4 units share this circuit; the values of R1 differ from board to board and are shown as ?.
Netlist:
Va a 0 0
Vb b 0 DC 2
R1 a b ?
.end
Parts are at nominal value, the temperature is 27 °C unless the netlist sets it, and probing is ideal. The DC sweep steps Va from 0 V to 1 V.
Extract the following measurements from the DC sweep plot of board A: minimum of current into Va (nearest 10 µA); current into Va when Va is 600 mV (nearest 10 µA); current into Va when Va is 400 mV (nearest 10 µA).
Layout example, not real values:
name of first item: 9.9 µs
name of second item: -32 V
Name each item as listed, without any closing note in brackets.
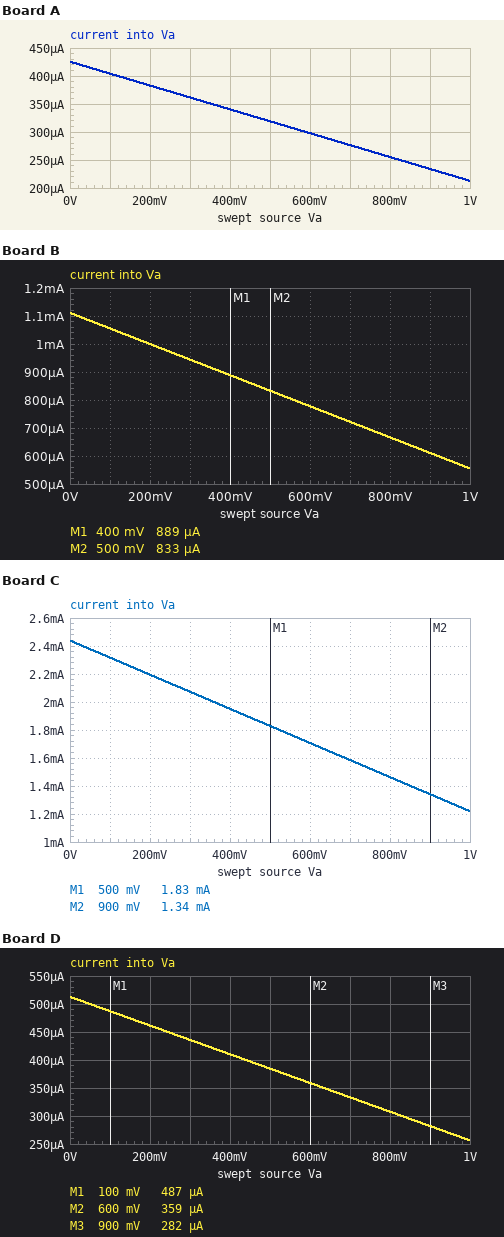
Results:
minimum of current into Va: 210 µA
current into Va when Va is 600 mV: 300 µA
current into Va when Va is 400 mV: 340 µA
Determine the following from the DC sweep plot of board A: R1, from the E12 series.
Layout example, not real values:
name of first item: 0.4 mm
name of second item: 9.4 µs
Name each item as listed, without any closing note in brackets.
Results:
R1, from the E12 series: 4.7 kΩ
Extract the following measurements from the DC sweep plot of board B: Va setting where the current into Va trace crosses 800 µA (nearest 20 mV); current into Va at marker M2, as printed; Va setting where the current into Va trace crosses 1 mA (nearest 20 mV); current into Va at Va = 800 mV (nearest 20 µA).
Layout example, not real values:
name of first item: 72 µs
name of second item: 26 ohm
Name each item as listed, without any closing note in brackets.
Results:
Va setting where the current into Va trace crosses 800 µA: 560 mV
current into Va at marker M2, as printed: 833 µA
Va setting where the current into Va trace crosses 1 mA: 200 mV
current into Va at Va = 800 mV: 660 µA
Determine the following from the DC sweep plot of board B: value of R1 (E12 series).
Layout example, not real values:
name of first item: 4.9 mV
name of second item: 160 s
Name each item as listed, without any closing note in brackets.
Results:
value of R1: 1.8 kΩ
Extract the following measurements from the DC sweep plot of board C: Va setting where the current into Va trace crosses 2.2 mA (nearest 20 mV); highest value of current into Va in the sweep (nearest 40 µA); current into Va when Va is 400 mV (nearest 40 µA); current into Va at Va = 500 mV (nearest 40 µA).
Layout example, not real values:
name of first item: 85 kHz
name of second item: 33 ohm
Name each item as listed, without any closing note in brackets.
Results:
Va setting where the current into Va trace crosses 2.2 mA: 200 mV
highest value of current into Va in the sweep: 2.44 mA
current into Va when Va is 400 mV: 1.96 mA
current into Va at Va = 500 mV: 1.84 mA
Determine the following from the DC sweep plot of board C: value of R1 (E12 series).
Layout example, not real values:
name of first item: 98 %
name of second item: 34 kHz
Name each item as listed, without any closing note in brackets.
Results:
value of R1: 820 Ω
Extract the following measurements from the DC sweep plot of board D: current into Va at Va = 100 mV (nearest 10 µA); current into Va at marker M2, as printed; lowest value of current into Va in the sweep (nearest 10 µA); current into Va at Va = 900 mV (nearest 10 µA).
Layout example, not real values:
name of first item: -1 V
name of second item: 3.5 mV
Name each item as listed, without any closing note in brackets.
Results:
current into Va at Va = 100 mV: 490 µA
current into Va at marker M2, as printed: 359 µA
lowest value of current into Va in the sweep: 260 µA
current into Va at Va = 900 mV: 280 µA
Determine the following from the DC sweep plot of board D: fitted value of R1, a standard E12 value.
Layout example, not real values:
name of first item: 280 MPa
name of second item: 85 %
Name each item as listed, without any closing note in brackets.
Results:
fitted value of R1, a standard E12 value: 3.9 kΩ
